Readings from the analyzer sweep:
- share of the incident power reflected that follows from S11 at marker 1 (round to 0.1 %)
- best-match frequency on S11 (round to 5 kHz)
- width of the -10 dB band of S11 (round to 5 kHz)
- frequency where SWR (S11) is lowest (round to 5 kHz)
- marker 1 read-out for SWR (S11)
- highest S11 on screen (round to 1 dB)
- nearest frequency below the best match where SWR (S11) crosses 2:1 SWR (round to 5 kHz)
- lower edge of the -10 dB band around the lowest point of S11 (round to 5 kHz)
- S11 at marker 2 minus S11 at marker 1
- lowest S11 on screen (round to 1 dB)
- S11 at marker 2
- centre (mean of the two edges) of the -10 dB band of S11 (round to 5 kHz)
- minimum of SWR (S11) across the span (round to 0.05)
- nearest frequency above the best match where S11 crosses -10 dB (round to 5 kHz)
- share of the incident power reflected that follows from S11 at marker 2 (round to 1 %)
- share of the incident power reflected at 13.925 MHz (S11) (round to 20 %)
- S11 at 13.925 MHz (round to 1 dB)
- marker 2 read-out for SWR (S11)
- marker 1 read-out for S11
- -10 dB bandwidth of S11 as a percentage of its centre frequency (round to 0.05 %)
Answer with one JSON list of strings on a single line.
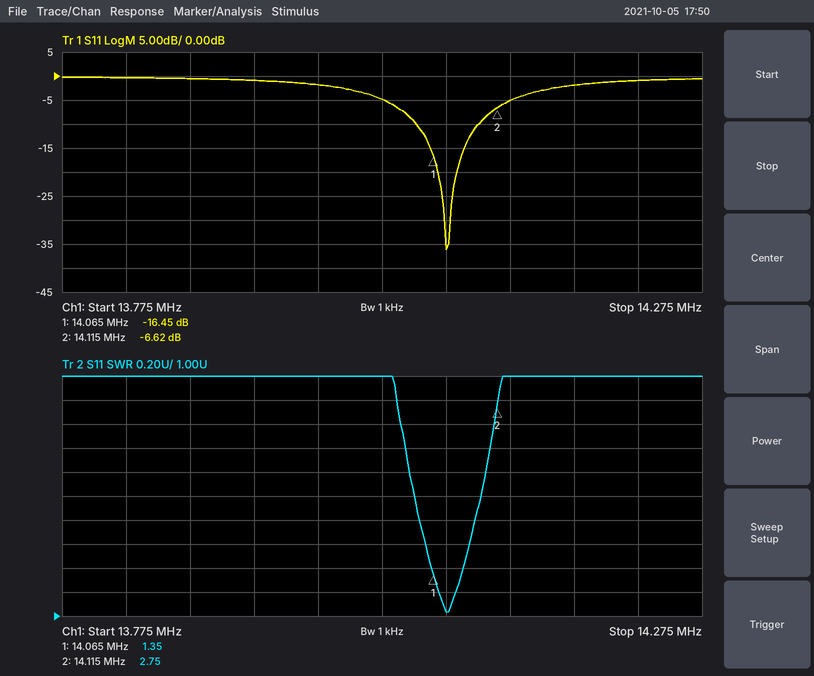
["2.3 %", "14.075 MHz", "50 kHz", "14.075 MHz", "1.35", "0 dB", "14.050 MHz", "14.050 MHz", "9.83 dB", "-36 dB", "-6.62 dB", "14.075 MHz", "1.05", "14.100 MHz", "22 %", "80 %", "-1 dB", "2.75", "-16.45 dB", "0.35 %"]
